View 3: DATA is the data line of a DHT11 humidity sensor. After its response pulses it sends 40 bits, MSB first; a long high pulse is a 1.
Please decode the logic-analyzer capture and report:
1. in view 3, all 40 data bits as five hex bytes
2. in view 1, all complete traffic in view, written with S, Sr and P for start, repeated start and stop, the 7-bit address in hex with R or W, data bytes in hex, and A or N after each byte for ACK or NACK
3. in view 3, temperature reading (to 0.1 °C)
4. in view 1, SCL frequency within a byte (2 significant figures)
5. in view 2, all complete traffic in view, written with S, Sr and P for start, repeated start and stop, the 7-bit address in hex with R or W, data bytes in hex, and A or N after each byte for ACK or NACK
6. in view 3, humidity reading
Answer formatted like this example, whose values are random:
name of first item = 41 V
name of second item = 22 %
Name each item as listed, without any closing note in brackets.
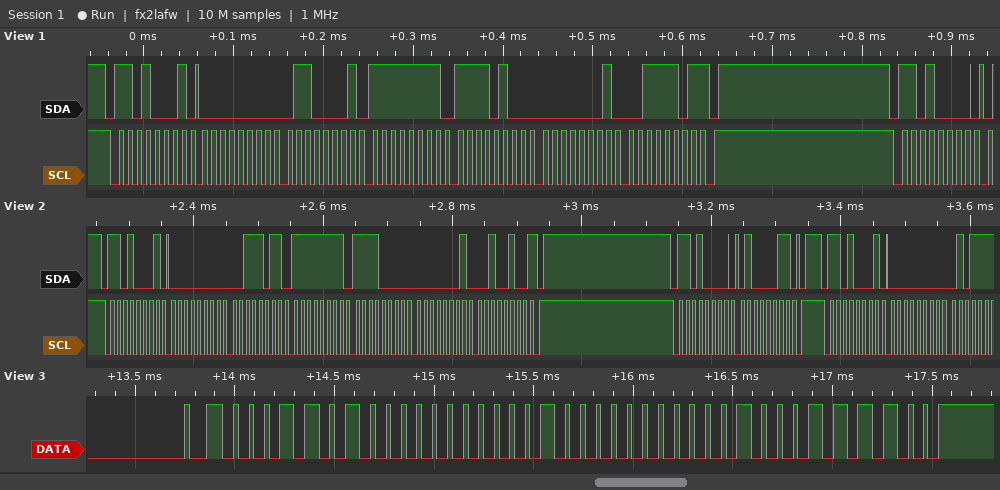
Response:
in view 3, all 40 data bits as five hex bytes = 1A 00 20 02 3C
in view 1, all complete traffic in view, written with S, Sr and P for start, repeated start and stop, the 7-bit address in hex with R or W, data bytes in hex, and A or N after each byte for ACK or NACK = S 68R A 00 A 61 A FF A F4 A 01 A 3D N P S 68W A
in view 3, temperature reading = 32.2 °C
in view 1, SCL frequency within a byte = 100 kHz
in view 2, all complete traffic in view, written with S, Sr and P for start, repeated start and stop, the 7-bit address in hex with R or W, data bytes in hex, and A or N after each byte for ACK or NACK = S 68R A 00 A 3B A FF A F0 A 01 A 24 N P S 68W A 43 A P S 68R A 00 A
in view 3, humidity reading = 26 %
